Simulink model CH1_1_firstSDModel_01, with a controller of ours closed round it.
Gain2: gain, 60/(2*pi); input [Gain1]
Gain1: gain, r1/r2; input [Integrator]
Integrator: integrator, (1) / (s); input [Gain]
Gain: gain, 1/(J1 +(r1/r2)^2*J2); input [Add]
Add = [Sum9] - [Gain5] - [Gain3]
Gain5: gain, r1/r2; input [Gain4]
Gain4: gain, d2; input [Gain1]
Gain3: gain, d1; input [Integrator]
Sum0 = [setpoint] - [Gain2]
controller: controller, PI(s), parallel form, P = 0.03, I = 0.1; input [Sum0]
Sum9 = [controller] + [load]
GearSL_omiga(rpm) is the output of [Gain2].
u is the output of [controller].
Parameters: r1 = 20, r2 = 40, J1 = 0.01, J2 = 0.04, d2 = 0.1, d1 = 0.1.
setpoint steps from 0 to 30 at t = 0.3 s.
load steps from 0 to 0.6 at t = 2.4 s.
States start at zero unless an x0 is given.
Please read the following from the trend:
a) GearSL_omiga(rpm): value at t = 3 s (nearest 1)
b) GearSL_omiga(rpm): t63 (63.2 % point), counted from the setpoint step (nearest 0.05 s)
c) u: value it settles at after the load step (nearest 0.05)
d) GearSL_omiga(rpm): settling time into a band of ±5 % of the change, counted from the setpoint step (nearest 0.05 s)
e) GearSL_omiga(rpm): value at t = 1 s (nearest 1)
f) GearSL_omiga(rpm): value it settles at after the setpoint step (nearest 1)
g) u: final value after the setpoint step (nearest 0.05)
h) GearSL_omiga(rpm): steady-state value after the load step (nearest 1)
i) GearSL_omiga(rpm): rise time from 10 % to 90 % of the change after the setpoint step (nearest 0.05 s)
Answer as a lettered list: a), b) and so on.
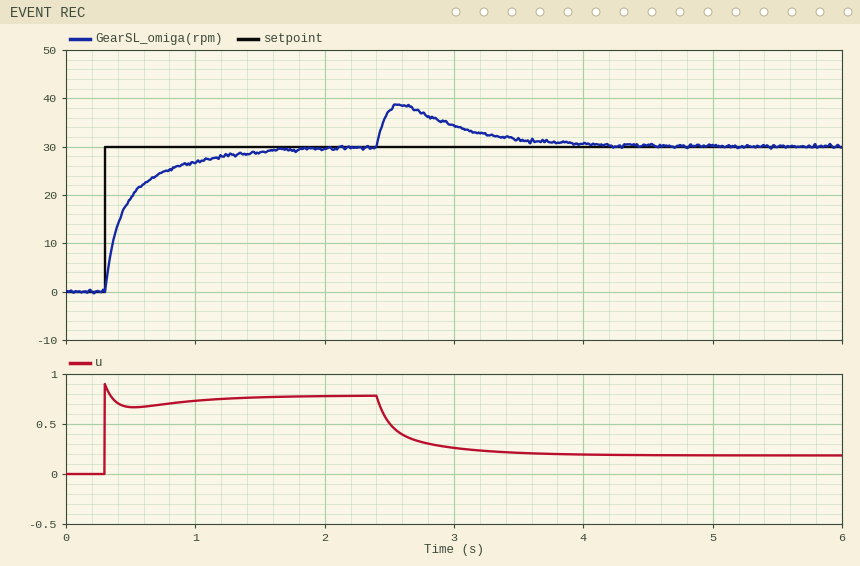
a) 34
b) 0.20 s
c) 0.20
d) 1.05 s
e) 27
f) 30
g) 0.80
h) 30
i) 0.70 s
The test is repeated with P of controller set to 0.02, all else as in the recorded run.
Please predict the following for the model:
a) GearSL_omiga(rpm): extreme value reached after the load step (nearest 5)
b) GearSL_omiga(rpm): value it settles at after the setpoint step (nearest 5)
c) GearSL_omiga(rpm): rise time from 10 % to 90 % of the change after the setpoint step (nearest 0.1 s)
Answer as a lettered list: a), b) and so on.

a) 40
b) 30
c) 0.6 s
